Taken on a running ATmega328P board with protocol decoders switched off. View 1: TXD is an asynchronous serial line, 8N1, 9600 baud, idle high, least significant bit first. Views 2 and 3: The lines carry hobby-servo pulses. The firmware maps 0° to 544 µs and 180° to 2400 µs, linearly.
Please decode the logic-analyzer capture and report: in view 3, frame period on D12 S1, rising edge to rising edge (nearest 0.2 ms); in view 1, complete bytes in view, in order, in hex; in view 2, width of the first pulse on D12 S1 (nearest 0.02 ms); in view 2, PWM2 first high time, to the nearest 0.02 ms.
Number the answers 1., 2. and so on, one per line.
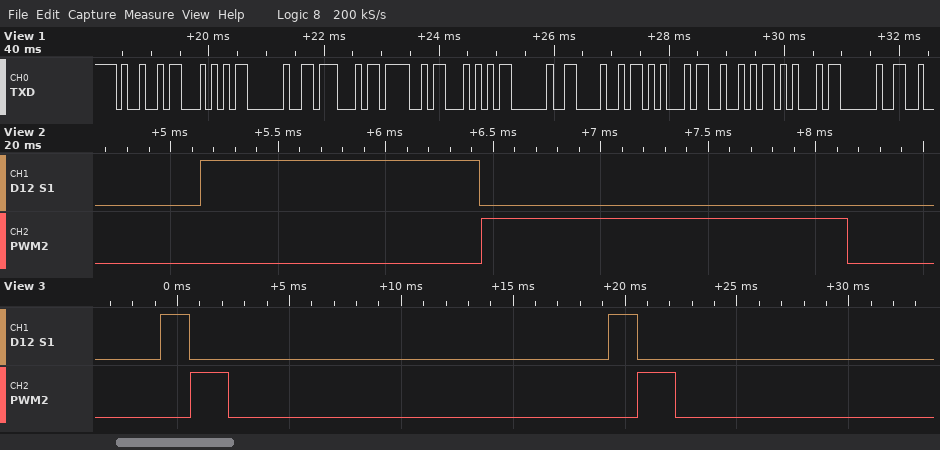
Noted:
1. 20.0 ms
2. 49 54 20 47 4F 54 20 48 45 52 45 20
3. 1.30 ms
4. 1.70 ms
